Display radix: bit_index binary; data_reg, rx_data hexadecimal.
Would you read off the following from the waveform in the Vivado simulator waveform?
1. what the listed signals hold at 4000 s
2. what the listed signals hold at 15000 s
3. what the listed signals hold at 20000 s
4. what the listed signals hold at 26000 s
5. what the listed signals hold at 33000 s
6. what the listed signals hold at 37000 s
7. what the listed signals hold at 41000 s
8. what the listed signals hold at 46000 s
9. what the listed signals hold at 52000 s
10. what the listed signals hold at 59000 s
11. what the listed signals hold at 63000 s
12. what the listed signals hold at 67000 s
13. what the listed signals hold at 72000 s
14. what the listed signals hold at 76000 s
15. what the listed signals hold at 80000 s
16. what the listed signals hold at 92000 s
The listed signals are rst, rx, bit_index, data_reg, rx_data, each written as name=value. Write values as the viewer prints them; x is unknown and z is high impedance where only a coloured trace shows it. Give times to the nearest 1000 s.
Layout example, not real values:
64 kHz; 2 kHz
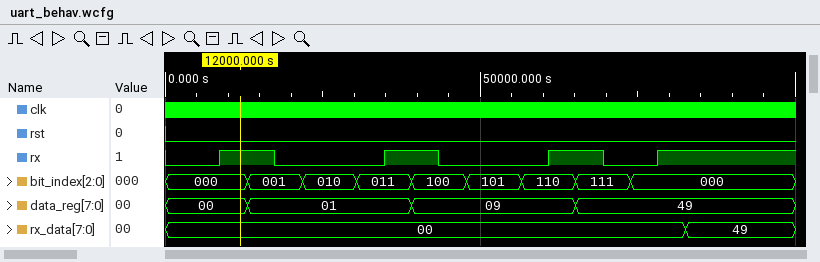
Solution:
rst=0, rx=0, bit_index=000, data_reg=00, rx_data=00; rst=0, rx=1, bit_index=001, data_reg=01, rx_data=00; rst=0, rx=0, bit_index=001, data_reg=01, rx_data=00; rst=0, rx=0, bit_index=010, data_reg=01, rx_data=00; rst=0, rx=0, bit_index=011, data_reg=01, rx_data=00; rst=0, rx=1, bit_index=011, data_reg=01, rx_data=00; rst=0, rx=1, bit_index=100, data_reg=09, rx_data=00; rst=0, rx=0, bit_index=100, data_reg=09, rx_data=00; rst=0, rx=0, bit_index=101, data_reg=09, rx_data=00; rst=0, rx=0, bit_index=110, data_reg=09, rx_data=00; rst=0, rx=1, bit_index=110, data_reg=09, rx_data=00; rst=0, rx=1, bit_index=111, data_reg=49, rx_data=00; rst=0, rx=0, bit_index=111, data_reg=49, rx_data=00; rst=0, rx=0, bit_index=000, data_reg=49, rx_data=00; rst=0, rx=1, bit_index=000, data_reg=49, rx_data=00; rst=0, rx=1, bit_index=000, data_reg=49, rx_data=49
